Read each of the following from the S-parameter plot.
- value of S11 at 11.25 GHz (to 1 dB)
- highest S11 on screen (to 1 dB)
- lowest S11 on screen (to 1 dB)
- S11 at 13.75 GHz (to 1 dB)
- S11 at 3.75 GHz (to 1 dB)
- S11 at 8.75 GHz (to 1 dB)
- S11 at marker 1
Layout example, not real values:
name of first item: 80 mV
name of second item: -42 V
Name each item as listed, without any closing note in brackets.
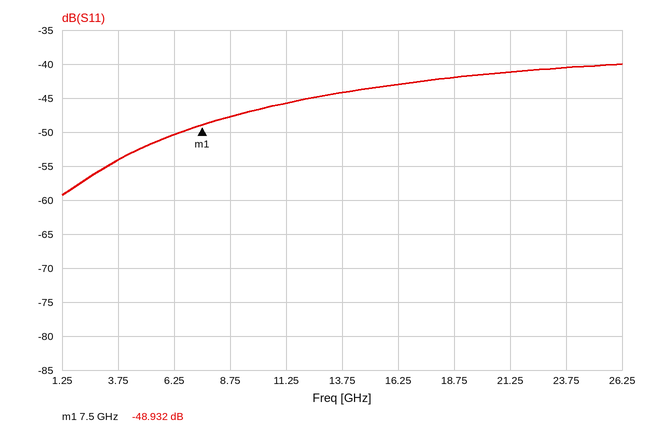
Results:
value of S11 at 11.25 GHz: -46 dB
highest S11 on screen: -40 dB
lowest S11 on screen: -59 dB
S11 at 13.75 GHz: -44 dB
S11 at 3.75 GHz: -54 dB
S11 at 8.75 GHz: -48 dB
S11 at marker 1: -48.932 dB
